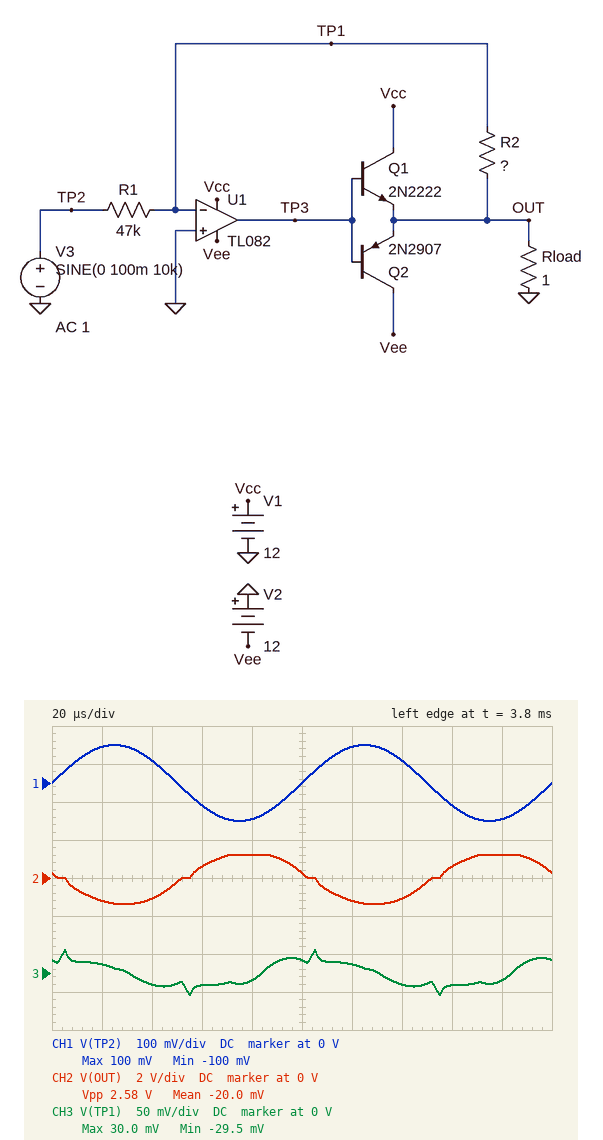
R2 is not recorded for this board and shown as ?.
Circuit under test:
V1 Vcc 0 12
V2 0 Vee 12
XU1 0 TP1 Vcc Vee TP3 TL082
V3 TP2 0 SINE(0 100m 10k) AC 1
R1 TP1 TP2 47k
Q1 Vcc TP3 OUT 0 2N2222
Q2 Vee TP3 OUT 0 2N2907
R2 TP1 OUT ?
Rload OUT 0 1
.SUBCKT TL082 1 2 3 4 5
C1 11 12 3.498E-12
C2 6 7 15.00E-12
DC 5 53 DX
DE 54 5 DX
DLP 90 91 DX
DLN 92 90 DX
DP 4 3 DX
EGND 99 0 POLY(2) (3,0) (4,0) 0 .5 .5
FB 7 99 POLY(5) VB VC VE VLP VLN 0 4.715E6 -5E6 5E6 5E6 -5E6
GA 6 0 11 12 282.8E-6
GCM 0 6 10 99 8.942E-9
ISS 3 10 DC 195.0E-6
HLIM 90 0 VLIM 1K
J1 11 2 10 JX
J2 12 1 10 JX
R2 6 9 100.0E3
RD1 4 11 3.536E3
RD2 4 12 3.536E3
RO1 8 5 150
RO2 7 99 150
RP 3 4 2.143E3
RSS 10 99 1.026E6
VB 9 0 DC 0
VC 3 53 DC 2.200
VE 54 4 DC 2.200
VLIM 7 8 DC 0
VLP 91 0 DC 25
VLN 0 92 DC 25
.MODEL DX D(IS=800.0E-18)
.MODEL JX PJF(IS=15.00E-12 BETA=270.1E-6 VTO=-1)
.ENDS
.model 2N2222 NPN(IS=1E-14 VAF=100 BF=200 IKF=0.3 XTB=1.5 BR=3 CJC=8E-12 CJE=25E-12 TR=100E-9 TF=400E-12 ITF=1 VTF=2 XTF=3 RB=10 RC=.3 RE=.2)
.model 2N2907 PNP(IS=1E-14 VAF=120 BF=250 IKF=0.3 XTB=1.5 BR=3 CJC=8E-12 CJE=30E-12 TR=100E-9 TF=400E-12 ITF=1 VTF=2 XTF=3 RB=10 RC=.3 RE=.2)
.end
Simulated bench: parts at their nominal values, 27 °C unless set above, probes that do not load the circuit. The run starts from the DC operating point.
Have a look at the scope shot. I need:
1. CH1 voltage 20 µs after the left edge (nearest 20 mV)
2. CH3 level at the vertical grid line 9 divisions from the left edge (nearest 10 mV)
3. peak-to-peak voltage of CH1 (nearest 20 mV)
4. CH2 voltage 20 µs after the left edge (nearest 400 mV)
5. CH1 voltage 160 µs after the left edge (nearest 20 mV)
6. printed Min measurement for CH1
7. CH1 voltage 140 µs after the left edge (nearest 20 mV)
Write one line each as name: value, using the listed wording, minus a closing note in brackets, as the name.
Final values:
CH1 voltage 20 µs after the left edge: 100 mV
CH3 level at the vertical grid line 9 divisions from the left edge: -10 mV
peak-to-peak voltage of CH1: 200 mV
CH2 voltage 20 µs after the left edge: -1.2 V
CH1 voltage 160 µs after the left edge: -60 mV
printed Min measurement for CH1: -100 mV
CH1 voltage 140 µs after the left edge: 60 mV
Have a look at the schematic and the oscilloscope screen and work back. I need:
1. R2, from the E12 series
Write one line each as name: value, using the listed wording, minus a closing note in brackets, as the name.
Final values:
R2, from the E12 series: 680 kΩ
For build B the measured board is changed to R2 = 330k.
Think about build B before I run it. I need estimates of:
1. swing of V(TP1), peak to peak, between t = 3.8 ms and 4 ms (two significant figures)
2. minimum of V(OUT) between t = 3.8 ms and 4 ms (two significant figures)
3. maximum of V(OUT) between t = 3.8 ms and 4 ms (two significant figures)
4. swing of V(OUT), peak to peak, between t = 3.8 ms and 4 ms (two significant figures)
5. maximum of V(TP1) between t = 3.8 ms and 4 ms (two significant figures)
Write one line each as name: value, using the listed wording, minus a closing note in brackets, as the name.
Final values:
swing of V(TP1), peak to peak, between t = 3.8 ms and 4 ms: 53 mV
minimum of V(OUT) between t = 3.8 ms and 4 ms: -700 mV
maximum of V(OUT) between t = 3.8 ms and 4 ms: 700 mV
swing of V(OUT), peak to peak, between t = 3.8 ms and 4 ms: 1.4 V
maximum of V(TP1) between t = 3.8 ms and 4 ms: 27 mV
